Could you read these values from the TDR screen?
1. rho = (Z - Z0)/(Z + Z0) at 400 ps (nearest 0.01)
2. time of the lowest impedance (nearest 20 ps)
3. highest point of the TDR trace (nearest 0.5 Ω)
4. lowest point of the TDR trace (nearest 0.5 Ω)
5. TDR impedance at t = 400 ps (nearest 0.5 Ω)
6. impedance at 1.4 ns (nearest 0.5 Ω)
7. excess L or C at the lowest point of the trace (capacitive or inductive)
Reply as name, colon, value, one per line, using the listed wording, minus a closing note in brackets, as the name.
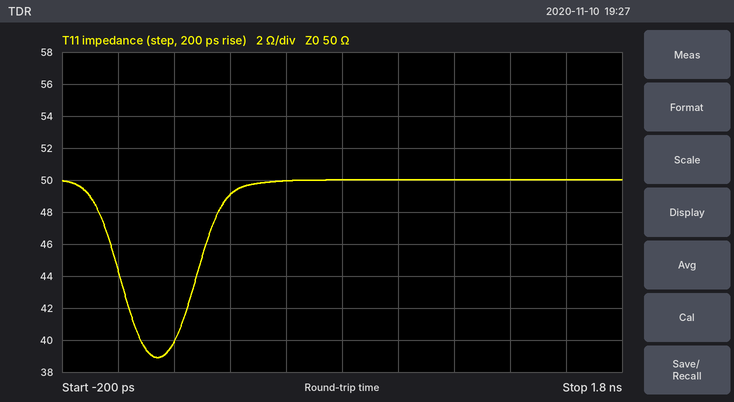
rho = (Z - Z0)/(Z + Z0) at 400 ps: -0.01
time of the lowest impedance: 140 ps
highest point of the TDR trace: 50.0 Ω
lowest point of the TDR trace: 39.0 Ω
TDR impedance at t = 400 ps: 49.0 Ω
impedance at 1.4 ns: 50.0 Ω
excess L or C at the lowest point of the trace: capacitive
